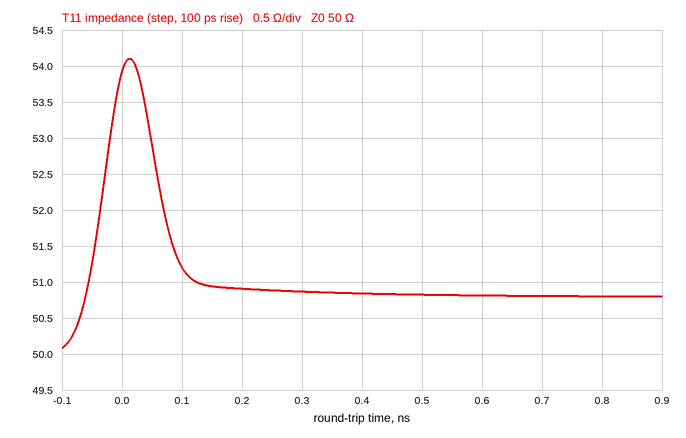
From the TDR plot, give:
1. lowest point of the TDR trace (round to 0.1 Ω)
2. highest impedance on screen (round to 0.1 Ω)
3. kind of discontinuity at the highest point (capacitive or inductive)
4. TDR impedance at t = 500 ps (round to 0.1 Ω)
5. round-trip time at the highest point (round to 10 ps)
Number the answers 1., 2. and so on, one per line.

1. 50.1 Ω
2. 54.1 Ω
3. inductive
4. 50.8 Ω
5. 10 ps
